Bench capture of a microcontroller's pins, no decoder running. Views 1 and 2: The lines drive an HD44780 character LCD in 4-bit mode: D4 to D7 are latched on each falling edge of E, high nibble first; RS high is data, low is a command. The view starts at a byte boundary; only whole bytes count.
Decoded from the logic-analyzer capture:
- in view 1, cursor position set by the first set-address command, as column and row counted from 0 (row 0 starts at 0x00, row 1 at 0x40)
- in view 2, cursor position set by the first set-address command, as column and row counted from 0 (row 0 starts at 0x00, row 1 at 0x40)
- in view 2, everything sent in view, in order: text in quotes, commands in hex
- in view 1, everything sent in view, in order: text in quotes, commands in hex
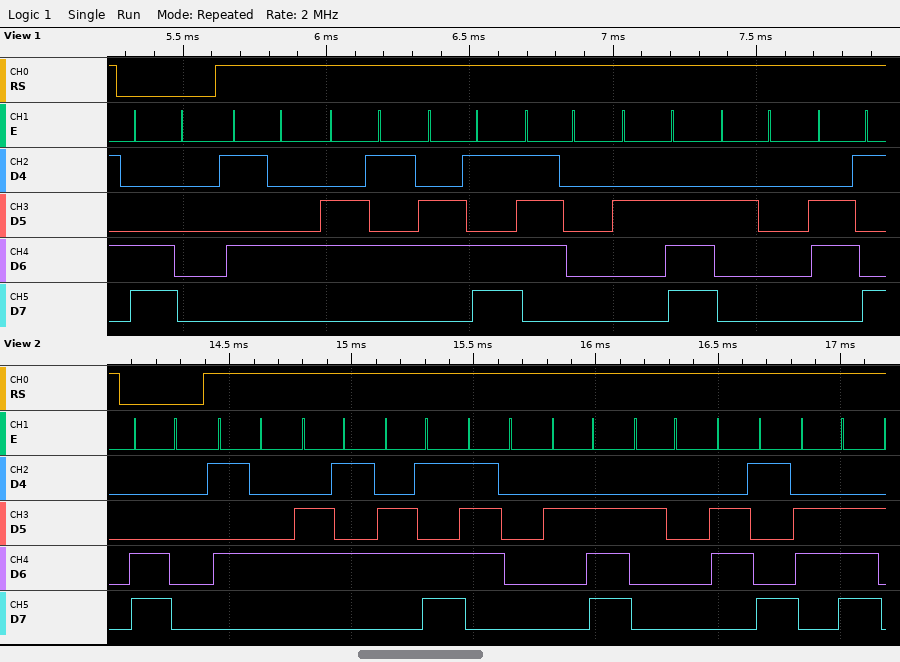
column 0, row 1
column 0, row 1
0xC0 "Temp. in"
0xC0 "Temp. i"
